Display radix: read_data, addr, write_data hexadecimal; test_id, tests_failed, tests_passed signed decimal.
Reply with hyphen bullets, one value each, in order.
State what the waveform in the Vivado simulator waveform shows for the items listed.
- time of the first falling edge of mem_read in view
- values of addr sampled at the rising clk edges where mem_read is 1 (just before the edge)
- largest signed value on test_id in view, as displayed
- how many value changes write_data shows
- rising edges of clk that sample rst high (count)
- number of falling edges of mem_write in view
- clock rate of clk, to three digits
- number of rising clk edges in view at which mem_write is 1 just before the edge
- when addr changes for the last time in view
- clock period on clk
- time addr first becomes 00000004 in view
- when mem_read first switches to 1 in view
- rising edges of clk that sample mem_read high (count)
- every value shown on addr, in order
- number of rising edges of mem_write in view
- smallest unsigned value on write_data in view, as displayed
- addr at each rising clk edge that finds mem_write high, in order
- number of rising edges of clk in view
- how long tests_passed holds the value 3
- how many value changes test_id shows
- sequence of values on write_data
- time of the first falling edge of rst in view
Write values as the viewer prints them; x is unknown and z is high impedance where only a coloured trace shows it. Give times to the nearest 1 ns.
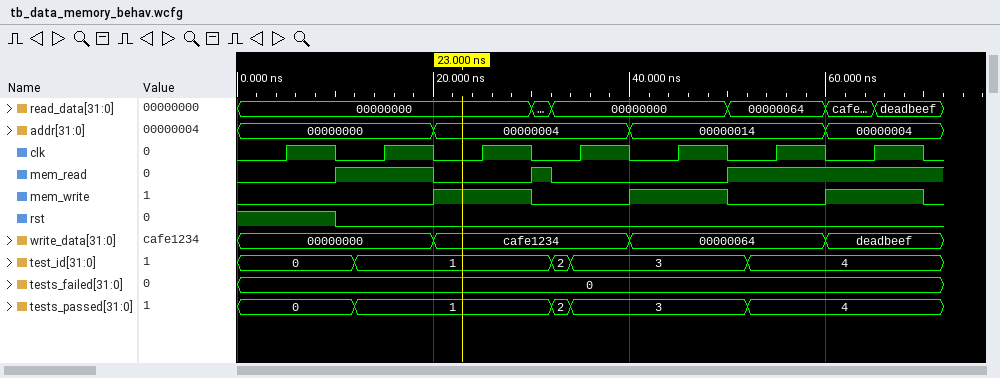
- 20 ns
- 00000000, 00000014, 00000004
- 4
- 3
- 1
- 3
- 100 MHz
- 3
- 60 ns
- 10 ns
- 20 ns
- 10 ns
- 3
- 00000000, 00000004, 00000014, 00000004
- 3
- 00000000
- 00000004, 00000014, 00000004
- 7
- 18 ns
- 4
- 00000000, cafe1234, 00000064, deadbeef
- 10 ns
